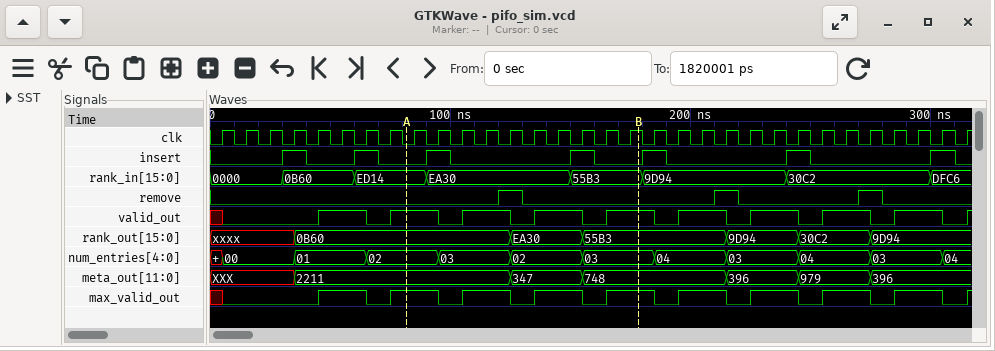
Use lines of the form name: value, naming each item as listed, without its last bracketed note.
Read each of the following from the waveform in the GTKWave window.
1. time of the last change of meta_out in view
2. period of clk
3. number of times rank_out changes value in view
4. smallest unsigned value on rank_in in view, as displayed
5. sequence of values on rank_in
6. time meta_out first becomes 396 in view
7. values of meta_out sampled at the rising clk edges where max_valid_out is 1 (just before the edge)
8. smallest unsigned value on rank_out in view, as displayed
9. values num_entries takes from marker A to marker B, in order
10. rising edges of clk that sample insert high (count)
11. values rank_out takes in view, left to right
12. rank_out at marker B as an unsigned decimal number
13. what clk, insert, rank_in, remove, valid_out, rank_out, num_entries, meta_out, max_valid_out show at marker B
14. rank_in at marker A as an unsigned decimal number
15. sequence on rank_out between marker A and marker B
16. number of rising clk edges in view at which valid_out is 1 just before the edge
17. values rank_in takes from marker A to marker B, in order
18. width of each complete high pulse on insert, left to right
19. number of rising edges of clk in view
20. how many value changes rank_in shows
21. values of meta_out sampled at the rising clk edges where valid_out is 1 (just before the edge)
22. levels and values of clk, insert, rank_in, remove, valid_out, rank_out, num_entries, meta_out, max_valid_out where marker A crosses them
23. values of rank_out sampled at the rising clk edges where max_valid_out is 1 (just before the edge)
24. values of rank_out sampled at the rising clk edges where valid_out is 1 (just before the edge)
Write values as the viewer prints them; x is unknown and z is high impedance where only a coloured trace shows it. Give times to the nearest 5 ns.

time of the last change of meta_out in view: 275 ns
period of clk: 10 ns
number of times rank_out changes value in view: 6
smallest unsigned value on rank_in in view, as displayed: 0000
sequence of values on rank_in: 0000, 0B60, ED14, EA30, 55B3, 9D94, 30C2, DFC6
time meta_out first becomes 396 in view: 215 ns
values of meta_out sampled at the rising clk edges where max_valid_out is 1: 2211, 2211, 2211, 2211, 2211, 2211, 347, 347, 748, 748, 748, 748, 396, 396, 979, 979, 396, 396
smallest unsigned value on rank_out in view, as displayed: 0B60
values num_entries takes from marker A to marker B, in order: 02, 03, 02, 03
rising edges of clk that sample insert high: 7
values rank_out takes in view, left to right: xxxx, 0B60, EA30, 55B3, 9D94, 30C2, 9D94
rank_out at marker B as an unsigned decimal number: 21939
what clk, insert, rank_in, remove, valid_out, rank_out, num_entries, meta_out, max_valid_out show at marker B: clk=1, insert=0, rank_in=55B3, remove=0, valid_out=1, rank_out=55B3, num_entries=03, meta_out=748, max_valid_out=1
rank_in at marker A as an unsigned decimal number: 60692
sequence on rank_out between marker A and marker B: 0B60, EA30, 55B3
number of rising clk edges in view at which valid_out is 1 just before the edge: 18
values rank_in takes from marker A to marker B, in order: ED14, EA30, 55B3
width of each complete high pulse on insert, left to right: 10 ns, 10 ns, 10 ns, 10 ns, 10 ns, 10 ns, 10 ns
number of rising edges of clk in view: 32
how many value changes rank_in shows: 7
values of meta_out sampled at the rising clk edges where valid_out is 1: 2211, 2211, 2211, 2211, 2211, 2211, 347, 347, 748, 748, 748, 748, 396, 396, 979, 979, 396, 396
levels and values of clk, insert, rank_in, remove, valid_out, rank_out, num_entries, meta_out, max_valid_out where marker A crosses them: clk=0, insert=0, rank_in=ED14, remove=0, valid_out=1, rank_out=0B60, num_entries=02, meta_out=2211, max_valid_out=1
values of rank_out sampled at the rising clk edges where max_valid_out is 1: 0B60, 0B60, 0B60, 0B60, 0B60, 0B60, EA30, EA30, 55B3, 55B3, 55B3, 55B3, 9D94, 9D94, 30C2, 30C2, 9D94, 9D94
values of rank_out sampled at the rising clk edges where valid_out is 1: 0B60, 0B60, 0B60, 0B60, 0B60, 0B60, EA30, EA30, 55B3, 55B3, 55B3, 55B3, 9D94, 9D94, 30C2, 30C2, 9D94, 9D94
